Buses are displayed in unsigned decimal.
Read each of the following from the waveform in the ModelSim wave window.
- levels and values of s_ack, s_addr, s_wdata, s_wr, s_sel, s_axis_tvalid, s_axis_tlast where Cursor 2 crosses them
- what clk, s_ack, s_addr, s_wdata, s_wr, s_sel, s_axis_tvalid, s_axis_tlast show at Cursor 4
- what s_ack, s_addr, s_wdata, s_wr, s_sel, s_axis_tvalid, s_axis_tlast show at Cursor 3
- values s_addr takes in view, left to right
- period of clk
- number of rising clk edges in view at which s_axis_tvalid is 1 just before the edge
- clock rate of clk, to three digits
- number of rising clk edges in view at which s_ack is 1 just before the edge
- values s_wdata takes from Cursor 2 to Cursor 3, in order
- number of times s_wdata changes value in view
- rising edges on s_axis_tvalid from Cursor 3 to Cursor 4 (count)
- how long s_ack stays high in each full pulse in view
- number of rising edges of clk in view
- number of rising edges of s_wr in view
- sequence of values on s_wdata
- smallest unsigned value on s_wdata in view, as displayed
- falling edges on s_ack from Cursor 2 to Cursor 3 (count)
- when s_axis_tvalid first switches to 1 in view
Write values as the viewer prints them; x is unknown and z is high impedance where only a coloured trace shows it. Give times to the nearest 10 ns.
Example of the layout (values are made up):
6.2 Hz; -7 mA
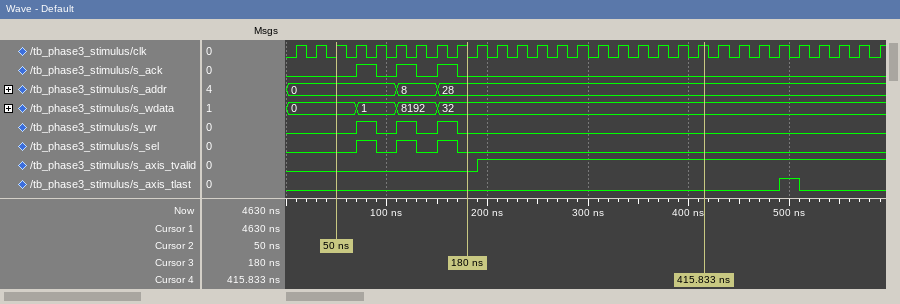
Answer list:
s_ack=0, s_addr=0, s_wdata=0, s_wr=0, s_sel=0, s_axis_tvalid=0, s_axis_tlast=0; clk=1, s_ack=0, s_addr=28, s_wdata=32, s_wr=0, s_sel=0, s_axis_tvalid=1, s_axis_tlast=0; s_ack=0, s_addr=28, s_wdata=32, s_wr=0, s_sel=0, s_axis_tvalid=0, s_axis_tlast=0; 0, 8, 28; 20 ns; 20; 50.0 MHz; 3; 0, 1, 8192, 32; 3; 1; 20 ns, 20 ns, 20 ns; 30; 3; 0, 1, 8192, 32; 0; 3; 190 ns
